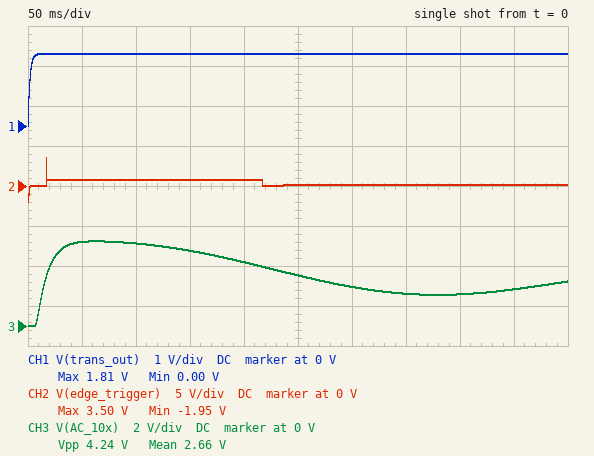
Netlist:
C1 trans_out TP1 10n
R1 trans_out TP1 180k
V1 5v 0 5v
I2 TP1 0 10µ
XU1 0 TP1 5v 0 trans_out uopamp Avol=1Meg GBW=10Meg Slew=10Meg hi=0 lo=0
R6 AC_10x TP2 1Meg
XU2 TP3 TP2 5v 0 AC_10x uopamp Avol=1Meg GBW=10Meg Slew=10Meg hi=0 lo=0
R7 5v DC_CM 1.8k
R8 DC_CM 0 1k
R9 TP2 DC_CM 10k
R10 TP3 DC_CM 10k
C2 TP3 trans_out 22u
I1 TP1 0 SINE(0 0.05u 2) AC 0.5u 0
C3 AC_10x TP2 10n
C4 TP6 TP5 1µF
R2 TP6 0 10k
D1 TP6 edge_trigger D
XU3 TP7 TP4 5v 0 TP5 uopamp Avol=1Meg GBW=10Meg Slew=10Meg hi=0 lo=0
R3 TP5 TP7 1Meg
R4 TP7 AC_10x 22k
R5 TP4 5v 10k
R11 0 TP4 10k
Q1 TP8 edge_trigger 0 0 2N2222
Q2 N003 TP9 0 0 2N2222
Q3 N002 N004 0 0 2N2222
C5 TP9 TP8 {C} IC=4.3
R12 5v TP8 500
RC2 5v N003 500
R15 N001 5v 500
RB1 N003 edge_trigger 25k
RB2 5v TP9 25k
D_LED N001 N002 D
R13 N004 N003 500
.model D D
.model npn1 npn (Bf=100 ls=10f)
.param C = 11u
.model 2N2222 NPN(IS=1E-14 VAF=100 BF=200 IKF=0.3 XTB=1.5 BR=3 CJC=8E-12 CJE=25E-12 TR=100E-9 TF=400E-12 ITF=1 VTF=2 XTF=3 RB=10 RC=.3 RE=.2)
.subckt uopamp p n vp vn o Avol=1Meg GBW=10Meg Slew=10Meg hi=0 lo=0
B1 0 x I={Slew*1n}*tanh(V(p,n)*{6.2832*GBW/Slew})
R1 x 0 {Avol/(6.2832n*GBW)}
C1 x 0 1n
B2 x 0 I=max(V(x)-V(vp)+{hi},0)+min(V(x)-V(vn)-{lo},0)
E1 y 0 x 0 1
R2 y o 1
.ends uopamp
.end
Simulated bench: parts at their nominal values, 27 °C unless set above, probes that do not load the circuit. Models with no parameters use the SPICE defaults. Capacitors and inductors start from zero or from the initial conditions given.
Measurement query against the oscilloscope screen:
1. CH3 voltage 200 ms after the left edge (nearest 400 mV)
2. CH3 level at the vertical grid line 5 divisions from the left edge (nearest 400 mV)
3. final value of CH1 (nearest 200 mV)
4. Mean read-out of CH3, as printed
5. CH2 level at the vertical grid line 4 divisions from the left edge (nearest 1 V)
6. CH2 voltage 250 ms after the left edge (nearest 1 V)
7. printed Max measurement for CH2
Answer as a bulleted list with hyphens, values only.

- 3.2 V
- 2.4 V
- 1.8 V
- 2.66 V
- 1 V
- 0 V
- 3.50 V
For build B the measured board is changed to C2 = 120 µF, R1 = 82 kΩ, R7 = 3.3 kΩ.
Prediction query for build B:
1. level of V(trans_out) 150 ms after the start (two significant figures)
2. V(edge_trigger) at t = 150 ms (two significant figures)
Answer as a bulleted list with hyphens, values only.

- 820 mV
- 93 mV
